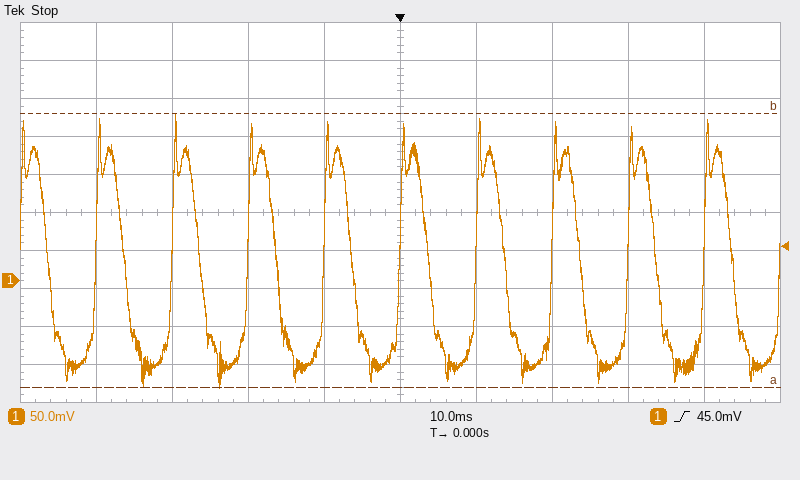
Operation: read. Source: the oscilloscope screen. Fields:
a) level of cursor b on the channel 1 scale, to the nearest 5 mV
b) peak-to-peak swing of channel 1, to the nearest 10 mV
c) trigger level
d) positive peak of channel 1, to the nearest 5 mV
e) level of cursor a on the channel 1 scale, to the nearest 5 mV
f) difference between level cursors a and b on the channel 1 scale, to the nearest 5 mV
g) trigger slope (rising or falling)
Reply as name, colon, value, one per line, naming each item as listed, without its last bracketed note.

level of cursor b on the channel 1 scale, to the nearest 5 mV: 220 mV
peak-to-peak swing of channel 1, to the nearest 10 mV: 360 mV
trigger level: 45.0 mV
positive peak of channel 1, to the nearest 5 mV: 220 mV
level of cursor a on the channel 1 scale, to the nearest 5 mV: -140 mV
difference between level cursors a and b on the channel 1 scale, to the nearest 5 mV: 360 mV
trigger slope: rising
